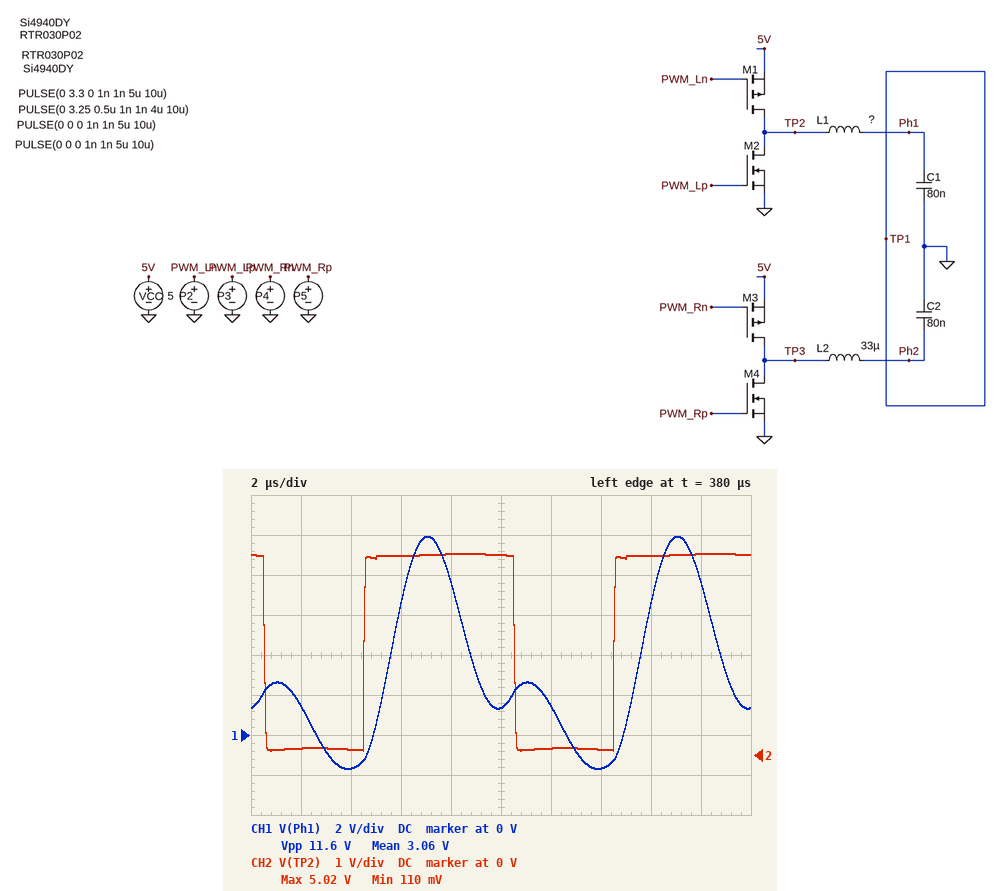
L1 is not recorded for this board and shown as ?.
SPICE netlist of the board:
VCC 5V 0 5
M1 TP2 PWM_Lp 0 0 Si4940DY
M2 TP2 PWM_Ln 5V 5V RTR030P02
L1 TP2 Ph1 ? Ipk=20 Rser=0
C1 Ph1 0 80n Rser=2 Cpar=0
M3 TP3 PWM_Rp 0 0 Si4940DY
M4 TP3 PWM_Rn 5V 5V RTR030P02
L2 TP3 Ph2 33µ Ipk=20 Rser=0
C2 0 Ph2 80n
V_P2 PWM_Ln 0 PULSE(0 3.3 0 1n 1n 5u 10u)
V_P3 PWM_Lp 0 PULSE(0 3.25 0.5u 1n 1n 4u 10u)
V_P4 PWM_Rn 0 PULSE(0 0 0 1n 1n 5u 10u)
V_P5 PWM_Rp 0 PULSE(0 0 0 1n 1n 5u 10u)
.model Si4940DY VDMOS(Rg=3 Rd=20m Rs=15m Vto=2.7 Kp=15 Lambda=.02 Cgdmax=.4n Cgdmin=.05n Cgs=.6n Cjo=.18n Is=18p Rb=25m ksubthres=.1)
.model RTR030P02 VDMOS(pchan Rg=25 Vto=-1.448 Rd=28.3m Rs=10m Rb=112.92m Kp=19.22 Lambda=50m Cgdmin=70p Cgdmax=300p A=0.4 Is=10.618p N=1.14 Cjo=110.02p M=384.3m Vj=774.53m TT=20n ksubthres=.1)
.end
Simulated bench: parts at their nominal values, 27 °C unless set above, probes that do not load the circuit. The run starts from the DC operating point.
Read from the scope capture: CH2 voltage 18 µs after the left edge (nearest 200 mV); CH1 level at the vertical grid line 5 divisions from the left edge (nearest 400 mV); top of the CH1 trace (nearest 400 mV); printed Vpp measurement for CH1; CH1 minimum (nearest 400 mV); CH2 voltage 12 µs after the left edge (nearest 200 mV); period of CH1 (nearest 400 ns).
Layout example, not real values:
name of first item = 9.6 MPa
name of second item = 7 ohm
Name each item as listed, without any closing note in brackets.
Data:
CH2 voltage 18 µs after the left edge = 5.0 V
CH1 level at the vertical grid line 5 divisions from the left edge = 1.2 V
top of the CH1 trace = 10.0 V
printed Vpp measurement for CH1 = 11.6 V
CH1 minimum = -1.6 V
CH2 voltage 12 µs after the left edge = 200 mV
period of CH1 = 10.0 µs
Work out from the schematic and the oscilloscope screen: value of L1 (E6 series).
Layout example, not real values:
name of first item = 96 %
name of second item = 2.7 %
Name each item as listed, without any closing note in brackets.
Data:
value of L1 = 10 µH
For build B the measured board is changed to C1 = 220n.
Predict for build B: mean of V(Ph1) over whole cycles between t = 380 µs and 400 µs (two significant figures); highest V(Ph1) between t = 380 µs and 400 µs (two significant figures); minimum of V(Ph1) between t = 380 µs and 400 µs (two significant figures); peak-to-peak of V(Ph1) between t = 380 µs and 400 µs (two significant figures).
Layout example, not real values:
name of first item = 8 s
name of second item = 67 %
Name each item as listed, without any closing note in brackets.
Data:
mean of V(Ph1) over whole cycles between t = 380 µs and 400 µs = 3.2 V
highest V(Ph1) between t = 380 µs and 400 µs = 12 V
minimum of V(Ph1) between t = 380 µs and 400 µs = -6.3 V
peak-to-peak of V(Ph1) between t = 380 µs and 400 µs = 18 V
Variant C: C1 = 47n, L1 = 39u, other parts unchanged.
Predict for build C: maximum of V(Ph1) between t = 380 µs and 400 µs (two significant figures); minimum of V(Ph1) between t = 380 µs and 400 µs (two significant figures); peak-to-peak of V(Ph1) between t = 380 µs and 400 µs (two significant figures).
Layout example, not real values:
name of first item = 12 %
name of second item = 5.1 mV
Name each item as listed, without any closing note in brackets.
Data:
maximum of V(Ph1) between t = 380 µs and 400 µs = 14 V
minimum of V(Ph1) between t = 380 µs and 400 µs = -7.0 V
peak-to-peak of V(Ph1) between t = 380 µs and 400 µs = 21 V
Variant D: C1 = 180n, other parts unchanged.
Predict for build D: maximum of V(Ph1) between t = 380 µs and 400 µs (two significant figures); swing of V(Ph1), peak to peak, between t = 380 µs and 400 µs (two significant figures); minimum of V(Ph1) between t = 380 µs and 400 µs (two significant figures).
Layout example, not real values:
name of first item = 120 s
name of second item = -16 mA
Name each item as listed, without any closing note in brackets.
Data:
maximum of V(Ph1) between t = 380 µs and 400 µs = 11 V
swing of V(Ph1), peak to peak, between t = 380 µs and 400 µs = 16 V
minimum of V(Ph1) between t = 380 µs and 400 µs = -4.8 V
